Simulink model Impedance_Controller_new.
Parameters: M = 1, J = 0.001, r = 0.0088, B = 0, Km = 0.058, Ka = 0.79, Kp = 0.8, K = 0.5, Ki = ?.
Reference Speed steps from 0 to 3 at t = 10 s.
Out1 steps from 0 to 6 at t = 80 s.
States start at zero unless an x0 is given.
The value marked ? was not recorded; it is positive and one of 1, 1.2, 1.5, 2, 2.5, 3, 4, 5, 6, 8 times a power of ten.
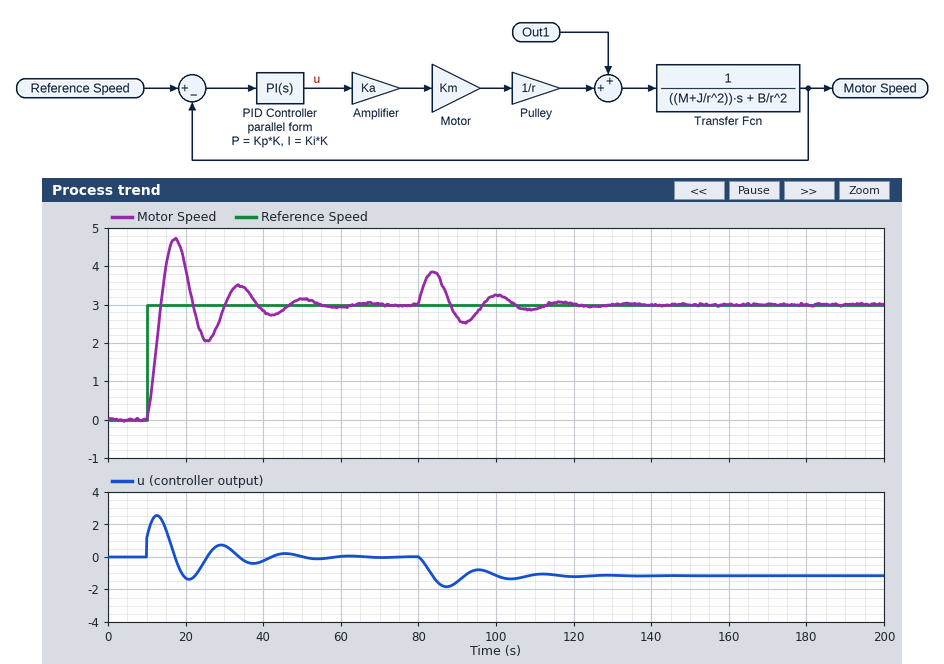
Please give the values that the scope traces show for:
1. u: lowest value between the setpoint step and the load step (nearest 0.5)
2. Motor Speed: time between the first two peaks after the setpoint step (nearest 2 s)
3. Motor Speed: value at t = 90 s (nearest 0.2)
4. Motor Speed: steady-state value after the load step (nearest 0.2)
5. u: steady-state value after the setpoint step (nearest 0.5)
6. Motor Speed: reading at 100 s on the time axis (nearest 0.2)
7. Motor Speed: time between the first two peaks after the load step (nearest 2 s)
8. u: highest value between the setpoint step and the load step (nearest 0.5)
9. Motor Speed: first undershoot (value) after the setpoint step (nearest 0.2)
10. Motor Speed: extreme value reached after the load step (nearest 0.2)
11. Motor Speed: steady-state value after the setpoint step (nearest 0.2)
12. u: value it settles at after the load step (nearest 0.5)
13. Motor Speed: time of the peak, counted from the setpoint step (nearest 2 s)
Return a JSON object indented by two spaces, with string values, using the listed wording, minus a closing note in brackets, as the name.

{
  "u: lowest value between the setpoint step and the load step": "-1.5",
  "Motor Speed: time between the first two peaks after the setpoint step": "16 s",
  "Motor Speed: value at t = 90 s": "2.6",
  "Motor Speed: steady-state value after the load step": "3.0",
  "u: steady-state value after the setpoint step": "0.0",
  "Motor Speed: reading at 100 s on the time axis": "3.2",
  "Motor Speed: time between the first two peaks after the load step": "16 s",
  "u: highest value between the setpoint step and the load step": "2.5",
  "Motor Speed: first undershoot (value) after the setpoint step": "2.0",
  "Motor Speed: extreme value reached after the load step": "3.8",
  "Motor Speed: steady-state value after the setpoint step": "3.0",
  "u: value it settles at after the load step": "-1.0",
  "Motor Speed: time of the peak, counted from the setpoint step": "8 s"
}
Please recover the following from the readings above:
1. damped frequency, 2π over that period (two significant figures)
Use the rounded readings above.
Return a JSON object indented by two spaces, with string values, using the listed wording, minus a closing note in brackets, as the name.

{
  "damped frequency, 2π over that period": "0.39 rad/s"
}
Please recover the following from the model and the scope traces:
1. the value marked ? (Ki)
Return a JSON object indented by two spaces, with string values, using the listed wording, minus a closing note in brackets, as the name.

{
  "the value marked ?": "0.8"
}
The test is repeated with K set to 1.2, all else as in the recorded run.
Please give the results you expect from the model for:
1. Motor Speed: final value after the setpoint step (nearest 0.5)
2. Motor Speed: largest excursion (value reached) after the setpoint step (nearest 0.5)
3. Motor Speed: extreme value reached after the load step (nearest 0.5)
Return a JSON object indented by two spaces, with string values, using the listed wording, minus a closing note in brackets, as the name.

{
  "Motor Speed: final value after the setpoint step": "3.0",
  "Motor Speed: largest excursion (value reached) after the setpoint step": "4.5",
  "Motor Speed: extreme value reached after the load step": "3.5"
}
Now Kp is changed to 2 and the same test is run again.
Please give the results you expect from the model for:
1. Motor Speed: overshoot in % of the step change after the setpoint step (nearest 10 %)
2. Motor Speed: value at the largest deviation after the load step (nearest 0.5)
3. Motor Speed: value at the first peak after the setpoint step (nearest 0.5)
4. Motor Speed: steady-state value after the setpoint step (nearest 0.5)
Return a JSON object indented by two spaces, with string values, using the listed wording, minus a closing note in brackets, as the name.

{
  "Motor Speed: overshoot in % of the step change after the setpoint step": "30 %",
  "Motor Speed: value at the largest deviation after the load step": "3.5",
  "Motor Speed: value at the first peak after the setpoint step": "4.0",
  "Motor Speed: steady-state value after the setpoint step": "3.0"
}
